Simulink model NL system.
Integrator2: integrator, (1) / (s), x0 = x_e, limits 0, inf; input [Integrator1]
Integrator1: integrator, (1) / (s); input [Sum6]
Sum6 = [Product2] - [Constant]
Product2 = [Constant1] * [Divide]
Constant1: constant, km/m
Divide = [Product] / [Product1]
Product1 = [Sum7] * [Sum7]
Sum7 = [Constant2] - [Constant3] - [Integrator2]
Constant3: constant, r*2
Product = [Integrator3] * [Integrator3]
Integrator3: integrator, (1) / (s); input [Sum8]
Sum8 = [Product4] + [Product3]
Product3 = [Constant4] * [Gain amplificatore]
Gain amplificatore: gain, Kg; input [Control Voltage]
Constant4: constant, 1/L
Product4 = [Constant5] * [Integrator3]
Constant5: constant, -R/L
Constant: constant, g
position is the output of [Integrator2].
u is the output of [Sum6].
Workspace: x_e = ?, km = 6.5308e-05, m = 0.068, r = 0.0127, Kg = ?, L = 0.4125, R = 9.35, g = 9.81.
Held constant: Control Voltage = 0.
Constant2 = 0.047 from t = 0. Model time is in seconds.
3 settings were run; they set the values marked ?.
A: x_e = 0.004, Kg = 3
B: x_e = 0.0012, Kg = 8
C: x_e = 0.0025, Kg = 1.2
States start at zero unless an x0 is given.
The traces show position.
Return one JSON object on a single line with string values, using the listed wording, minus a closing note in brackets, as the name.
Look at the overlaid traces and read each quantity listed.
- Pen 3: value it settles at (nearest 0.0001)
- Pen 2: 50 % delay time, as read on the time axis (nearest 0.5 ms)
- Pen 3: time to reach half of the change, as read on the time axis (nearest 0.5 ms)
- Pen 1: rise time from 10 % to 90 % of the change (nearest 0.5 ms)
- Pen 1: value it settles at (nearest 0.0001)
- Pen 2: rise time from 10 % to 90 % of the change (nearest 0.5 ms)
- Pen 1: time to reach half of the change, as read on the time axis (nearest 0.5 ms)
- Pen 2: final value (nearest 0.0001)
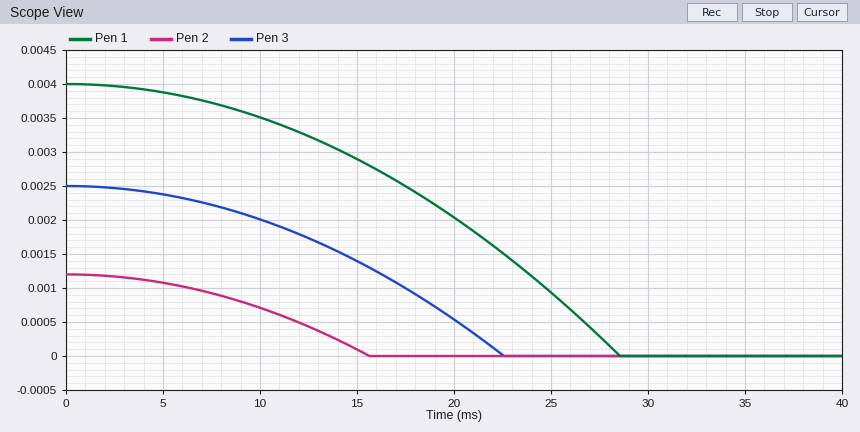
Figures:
{"Pen 3: value it settles at": "0.0000", "Pen 2: 50 % delay time, as read on the time axis": "11.0 ms", "Pen 3: time to reach half of the change, as read on the time axis": "16.0 ms", "Pen 1: rise time from 10 % to 90 % of the change": "18.0 ms", "Pen 1: value it settles at": "0.0000", "Pen 2: rise time from 10 % to 90 % of the change": "10.0 ms", "Pen 1: time to reach half of the change, as read on the time axis": "20.0 ms", "Pen 2: final value": "0.0000"}
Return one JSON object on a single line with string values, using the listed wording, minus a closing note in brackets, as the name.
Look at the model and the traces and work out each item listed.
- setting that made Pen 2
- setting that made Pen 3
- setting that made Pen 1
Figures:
{"setting that made Pen 2": "B", "setting that made Pen 3": "C", "setting that made Pen 1": "A"}
